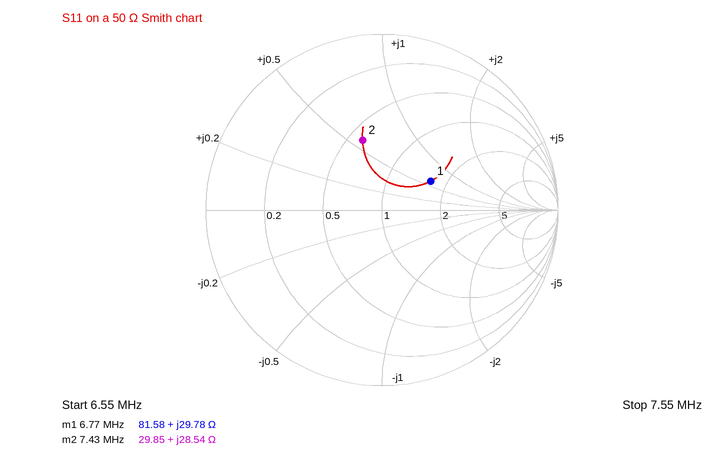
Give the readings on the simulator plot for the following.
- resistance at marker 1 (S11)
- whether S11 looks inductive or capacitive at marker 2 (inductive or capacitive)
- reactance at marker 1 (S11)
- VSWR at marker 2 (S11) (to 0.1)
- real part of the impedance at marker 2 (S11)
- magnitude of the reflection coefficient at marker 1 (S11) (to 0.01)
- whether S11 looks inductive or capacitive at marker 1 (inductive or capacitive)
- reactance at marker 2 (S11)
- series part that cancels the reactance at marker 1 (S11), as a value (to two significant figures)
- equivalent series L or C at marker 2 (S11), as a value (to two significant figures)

81.58 Ω
inductive
+29.78 Ω
2.4
29.85 Ω
0.32
inductive
+28.54 Ω
790 pF
610 nH
